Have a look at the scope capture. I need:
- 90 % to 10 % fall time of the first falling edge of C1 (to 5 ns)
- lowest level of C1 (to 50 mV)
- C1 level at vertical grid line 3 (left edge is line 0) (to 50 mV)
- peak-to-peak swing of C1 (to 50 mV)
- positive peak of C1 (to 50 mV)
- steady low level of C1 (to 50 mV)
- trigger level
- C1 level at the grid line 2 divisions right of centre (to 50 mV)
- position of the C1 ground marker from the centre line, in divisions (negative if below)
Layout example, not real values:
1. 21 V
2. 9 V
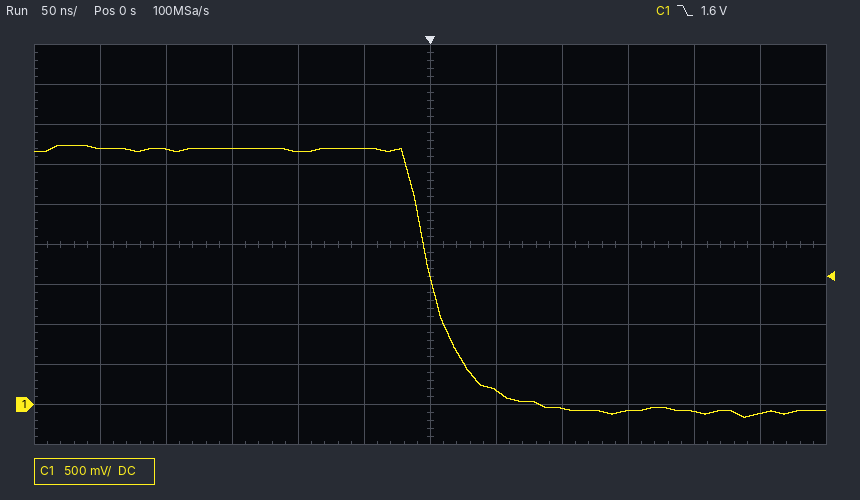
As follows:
1. 55 ns
2. -150 mV
3. 3.20 V
4. 3.40 V
5. 3.25 V
6. -100 mV
7. 1.6 V
8. -50 mV
9. -4.0 div
